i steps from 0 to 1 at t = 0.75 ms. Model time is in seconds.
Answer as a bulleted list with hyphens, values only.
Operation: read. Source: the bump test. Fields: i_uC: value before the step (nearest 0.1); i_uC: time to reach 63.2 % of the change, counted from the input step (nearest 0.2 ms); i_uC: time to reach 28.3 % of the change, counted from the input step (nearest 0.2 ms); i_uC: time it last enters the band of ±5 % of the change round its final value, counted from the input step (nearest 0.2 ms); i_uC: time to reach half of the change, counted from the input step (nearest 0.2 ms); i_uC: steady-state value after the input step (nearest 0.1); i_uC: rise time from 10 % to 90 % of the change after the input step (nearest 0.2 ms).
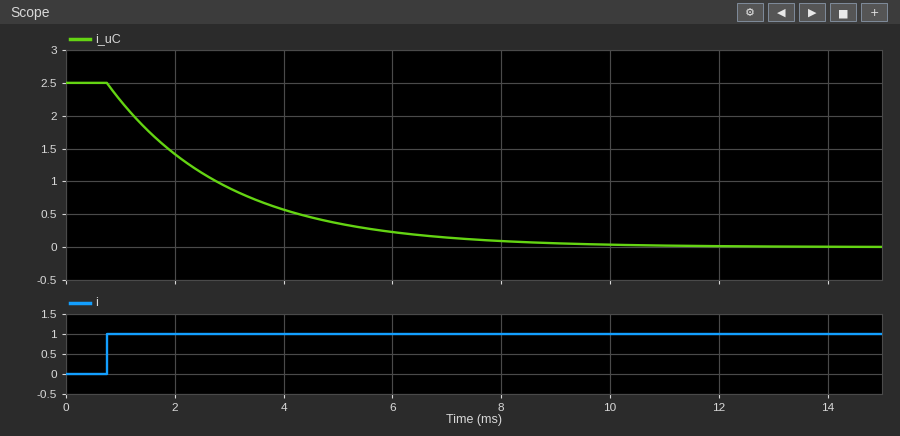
- 2.5
- 2.2 ms
- 0.8 ms
- 6.6 ms
- 1.6 ms
- 0.0
- 4.8 ms
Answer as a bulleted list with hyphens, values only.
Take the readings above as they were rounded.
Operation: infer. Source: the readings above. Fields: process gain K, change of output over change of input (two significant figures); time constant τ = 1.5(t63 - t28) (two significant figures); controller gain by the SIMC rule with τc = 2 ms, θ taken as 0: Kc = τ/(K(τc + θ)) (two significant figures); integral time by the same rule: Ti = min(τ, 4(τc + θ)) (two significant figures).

- -2.5
- 2.1 ms
- -0.42
- 2.1 ms
